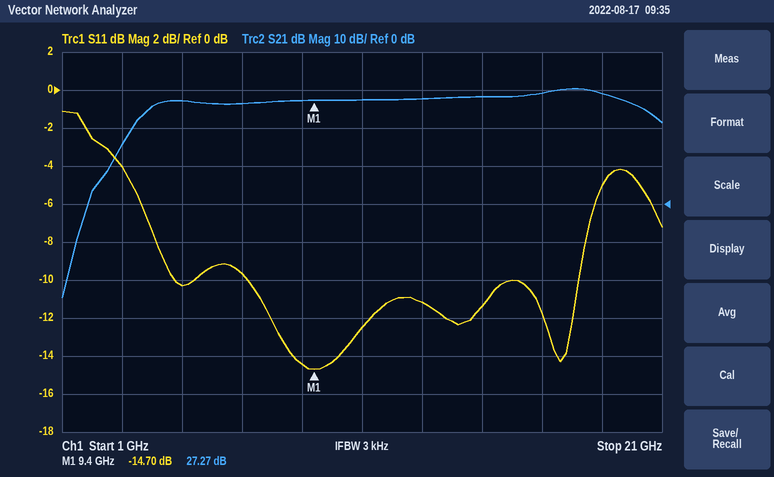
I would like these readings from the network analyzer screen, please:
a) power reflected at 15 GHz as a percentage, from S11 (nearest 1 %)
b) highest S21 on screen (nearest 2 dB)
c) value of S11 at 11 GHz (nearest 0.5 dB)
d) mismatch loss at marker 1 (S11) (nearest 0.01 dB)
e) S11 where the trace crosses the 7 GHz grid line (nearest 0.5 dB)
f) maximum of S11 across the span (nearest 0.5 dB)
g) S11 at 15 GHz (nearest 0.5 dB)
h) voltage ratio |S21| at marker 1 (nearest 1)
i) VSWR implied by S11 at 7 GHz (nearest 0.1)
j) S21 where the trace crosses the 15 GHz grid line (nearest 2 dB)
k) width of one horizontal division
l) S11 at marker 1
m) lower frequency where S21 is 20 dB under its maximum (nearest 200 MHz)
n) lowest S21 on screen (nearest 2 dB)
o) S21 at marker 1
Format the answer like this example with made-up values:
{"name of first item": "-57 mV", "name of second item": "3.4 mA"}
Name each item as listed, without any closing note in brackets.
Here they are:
{"power reflected at 15 GHz as a percentage, from S11": "7 %", "highest S21 on screen": "30 dB", "value of S11 at 11 GHz": "-12.5 dB", "mismatch loss at marker 1 (S11)": "0.15 dB", "S11 where the trace crosses the 7 GHz grid line": "-9.5 dB", "maximum of S11 across the span": "-1.0 dB", "S11 at 15 GHz": "-11.5 dB", "voltage ratio |S21| at marker 1": "23", "VSWR implied by S11 at 7 GHz": "2.0", "S21 where the trace crosses the 15 GHz grid line": "28 dB", "width of one horizontal division": "2 GHz", "S11 at marker 1": "-14.70 dB", "lower frequency where S21 is 20 dB under its maximum": "2.6 GHz", "lowest S21 on screen": "-24 dB", "S21 at marker 1": "27.27 dB"}
